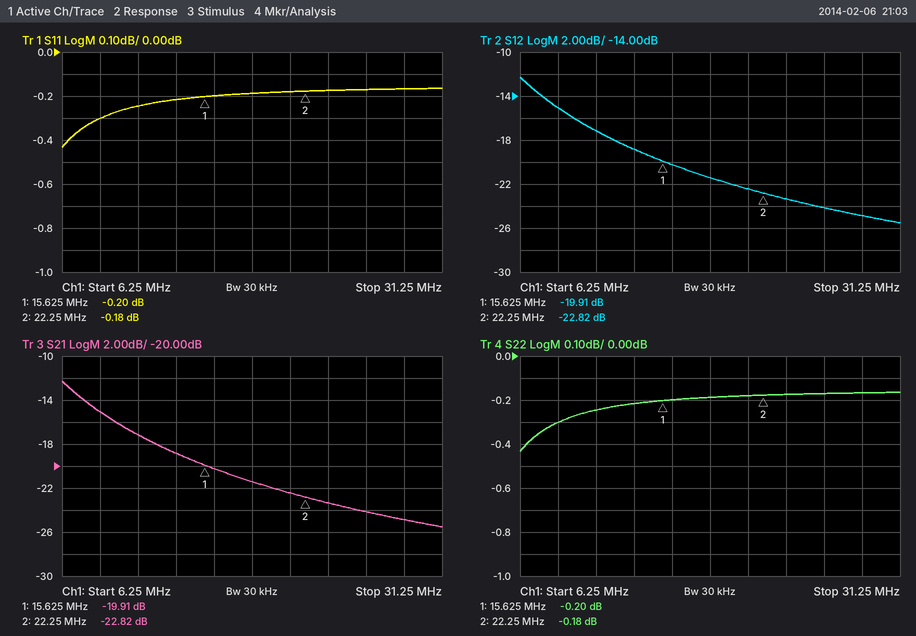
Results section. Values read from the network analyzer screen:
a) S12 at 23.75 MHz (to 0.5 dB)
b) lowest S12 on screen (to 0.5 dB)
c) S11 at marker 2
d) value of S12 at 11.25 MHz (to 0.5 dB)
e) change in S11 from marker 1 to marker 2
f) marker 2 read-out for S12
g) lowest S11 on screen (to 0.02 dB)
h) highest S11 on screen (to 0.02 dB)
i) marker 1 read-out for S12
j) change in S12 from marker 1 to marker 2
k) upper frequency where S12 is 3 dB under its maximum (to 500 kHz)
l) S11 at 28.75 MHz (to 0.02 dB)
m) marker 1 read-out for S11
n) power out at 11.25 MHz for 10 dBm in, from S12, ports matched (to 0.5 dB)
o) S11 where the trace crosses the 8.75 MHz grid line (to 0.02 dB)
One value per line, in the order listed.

-23.5 dB
-25.5 dB
-0.18 dB
-17.0 dB
0.02 dB
-22.82 dB
-0.44 dB
-0.16 dB
-19.91 dB
-2.91 dB
9.0 MHz
-0.16 dB
-0.20 dB
-7.0 dBm
-0.30 dB
